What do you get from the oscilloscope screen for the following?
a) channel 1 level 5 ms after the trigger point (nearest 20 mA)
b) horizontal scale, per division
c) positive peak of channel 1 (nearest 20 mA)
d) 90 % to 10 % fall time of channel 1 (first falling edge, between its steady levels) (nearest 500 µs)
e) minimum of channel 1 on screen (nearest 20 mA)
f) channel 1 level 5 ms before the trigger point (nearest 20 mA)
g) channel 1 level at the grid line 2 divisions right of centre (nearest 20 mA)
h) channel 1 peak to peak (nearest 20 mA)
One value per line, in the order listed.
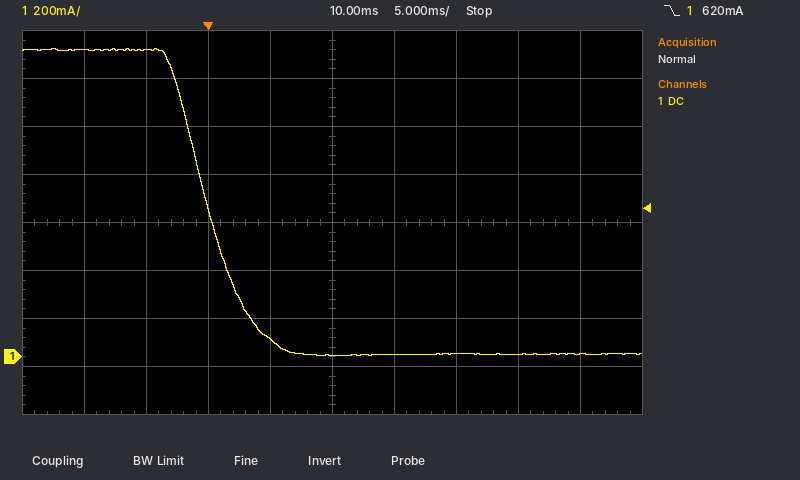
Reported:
80 mA
5 ms
1.28 A
6.5 ms
0 mA
1.28 A
20 mA
1.28 A
